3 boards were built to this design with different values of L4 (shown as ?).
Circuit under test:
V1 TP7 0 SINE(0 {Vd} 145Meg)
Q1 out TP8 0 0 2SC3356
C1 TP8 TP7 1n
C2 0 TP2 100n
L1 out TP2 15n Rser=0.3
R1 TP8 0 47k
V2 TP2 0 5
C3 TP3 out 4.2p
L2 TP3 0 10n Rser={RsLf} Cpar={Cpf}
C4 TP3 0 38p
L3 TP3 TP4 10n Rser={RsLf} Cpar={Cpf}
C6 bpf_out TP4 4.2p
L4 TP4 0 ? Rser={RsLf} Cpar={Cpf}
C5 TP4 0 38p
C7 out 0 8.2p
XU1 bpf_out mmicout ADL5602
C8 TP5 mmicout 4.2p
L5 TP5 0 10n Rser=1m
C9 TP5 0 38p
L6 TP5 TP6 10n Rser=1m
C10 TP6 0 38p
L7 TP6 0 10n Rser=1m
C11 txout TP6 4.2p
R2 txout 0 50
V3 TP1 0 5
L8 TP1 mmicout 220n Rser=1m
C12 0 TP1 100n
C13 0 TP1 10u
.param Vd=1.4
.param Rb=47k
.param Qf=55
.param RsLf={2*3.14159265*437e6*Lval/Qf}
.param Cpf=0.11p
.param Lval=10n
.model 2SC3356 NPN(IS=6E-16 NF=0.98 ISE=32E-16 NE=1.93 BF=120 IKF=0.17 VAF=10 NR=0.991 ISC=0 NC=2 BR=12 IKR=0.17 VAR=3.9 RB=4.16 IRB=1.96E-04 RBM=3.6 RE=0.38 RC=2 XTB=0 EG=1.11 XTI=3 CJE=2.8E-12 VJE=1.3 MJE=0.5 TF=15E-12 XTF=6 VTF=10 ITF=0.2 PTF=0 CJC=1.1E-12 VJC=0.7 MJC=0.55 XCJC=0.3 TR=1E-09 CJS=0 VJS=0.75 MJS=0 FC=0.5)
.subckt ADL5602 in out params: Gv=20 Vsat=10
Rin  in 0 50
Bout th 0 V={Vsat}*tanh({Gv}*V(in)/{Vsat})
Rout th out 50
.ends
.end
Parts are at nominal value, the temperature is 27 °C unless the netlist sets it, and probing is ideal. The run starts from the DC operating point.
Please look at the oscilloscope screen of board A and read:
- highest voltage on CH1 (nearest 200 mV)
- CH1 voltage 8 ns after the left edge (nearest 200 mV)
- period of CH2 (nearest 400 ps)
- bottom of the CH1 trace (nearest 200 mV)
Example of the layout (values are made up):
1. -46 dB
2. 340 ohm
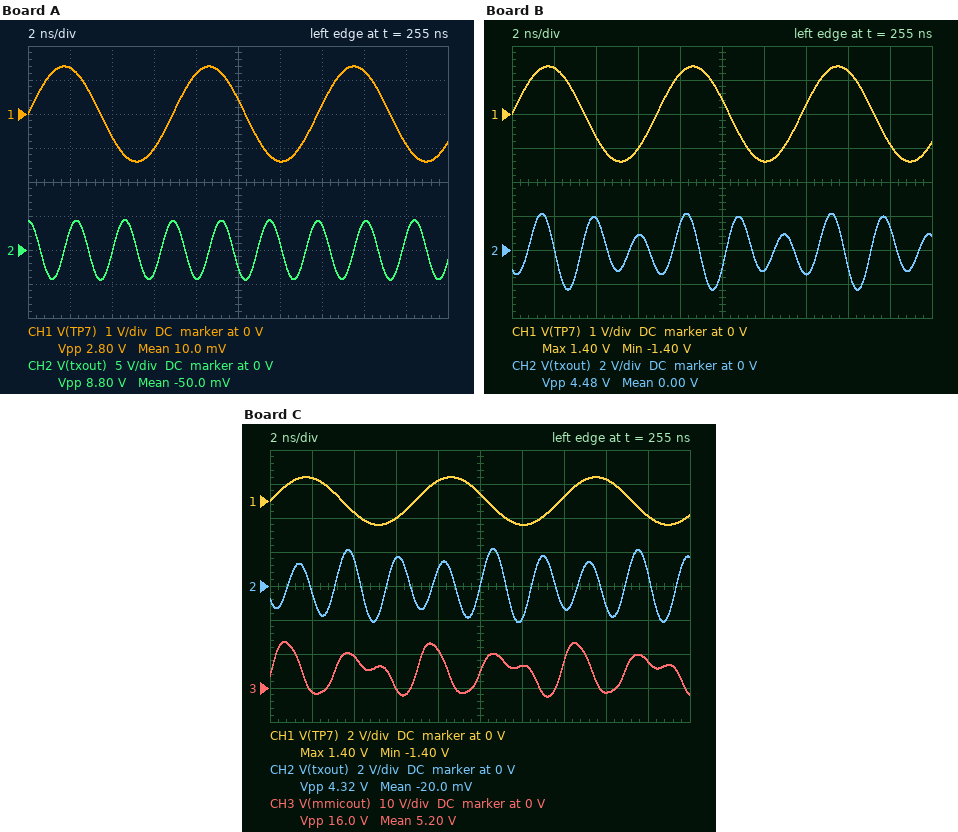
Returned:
1. 1.4 V
2. 1.2 V
3. 2.4 ns
4. -1.4 V
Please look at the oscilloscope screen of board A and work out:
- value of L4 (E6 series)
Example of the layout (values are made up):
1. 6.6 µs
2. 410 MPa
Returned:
1. 22 nH
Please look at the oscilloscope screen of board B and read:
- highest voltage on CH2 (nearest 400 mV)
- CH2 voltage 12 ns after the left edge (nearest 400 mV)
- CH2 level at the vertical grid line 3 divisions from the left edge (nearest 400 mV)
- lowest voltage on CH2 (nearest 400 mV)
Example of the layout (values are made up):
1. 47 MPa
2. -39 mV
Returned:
1. 2.0 V
2. -1.2 V
3. 800 mV
4. -2.4 V
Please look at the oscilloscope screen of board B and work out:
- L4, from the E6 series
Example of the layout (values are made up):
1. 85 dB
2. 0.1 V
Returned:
1. 4.7 nH
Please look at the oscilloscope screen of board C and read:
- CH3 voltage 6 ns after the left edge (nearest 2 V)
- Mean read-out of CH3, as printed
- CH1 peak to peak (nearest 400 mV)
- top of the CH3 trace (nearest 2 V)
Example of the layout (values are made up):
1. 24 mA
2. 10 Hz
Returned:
1. 0 V
2. 5.20 V
3. 2.8 V
4. 14 V
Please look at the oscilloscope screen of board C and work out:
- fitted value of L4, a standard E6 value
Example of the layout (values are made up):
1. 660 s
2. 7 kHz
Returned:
1. 3.3 nH
